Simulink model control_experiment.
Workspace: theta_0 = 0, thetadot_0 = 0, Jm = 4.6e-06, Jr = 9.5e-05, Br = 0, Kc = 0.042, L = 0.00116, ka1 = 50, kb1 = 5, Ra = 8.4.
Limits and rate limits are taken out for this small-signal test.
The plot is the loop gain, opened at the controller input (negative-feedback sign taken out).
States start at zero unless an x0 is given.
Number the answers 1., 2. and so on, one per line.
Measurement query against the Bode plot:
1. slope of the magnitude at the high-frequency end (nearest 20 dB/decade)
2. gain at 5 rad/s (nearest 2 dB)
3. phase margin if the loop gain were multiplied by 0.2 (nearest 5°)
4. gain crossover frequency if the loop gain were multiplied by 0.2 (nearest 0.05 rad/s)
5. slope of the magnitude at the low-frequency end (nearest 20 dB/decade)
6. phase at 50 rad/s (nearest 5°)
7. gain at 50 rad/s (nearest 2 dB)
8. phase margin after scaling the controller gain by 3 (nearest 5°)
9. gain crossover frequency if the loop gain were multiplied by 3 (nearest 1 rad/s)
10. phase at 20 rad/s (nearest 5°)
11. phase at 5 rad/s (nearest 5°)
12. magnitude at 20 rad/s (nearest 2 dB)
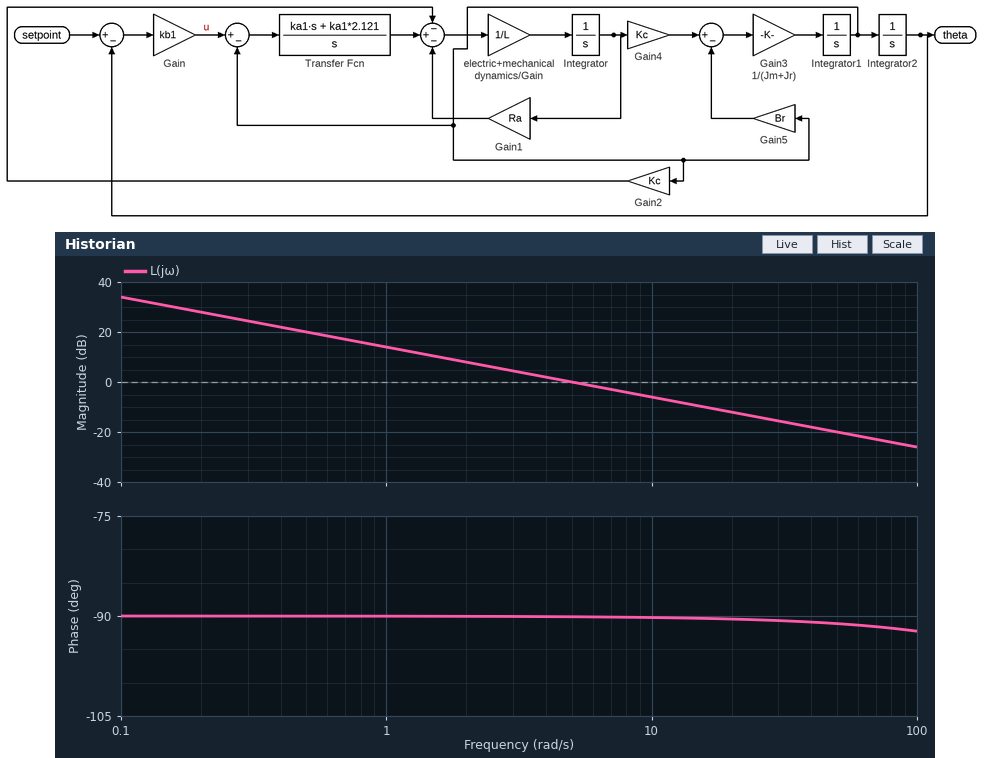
1. -20 dB/decade
2. 0 dB
3. 90°
4. 1.00 rad/s
5. -20 dB/decade
6. -90°
7. -20 dB
8. 90°
9. 15 rad/s
10. -90°
11. -90°
12. -12 dB
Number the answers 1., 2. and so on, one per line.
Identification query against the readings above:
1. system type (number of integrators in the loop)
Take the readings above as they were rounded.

1. 1
